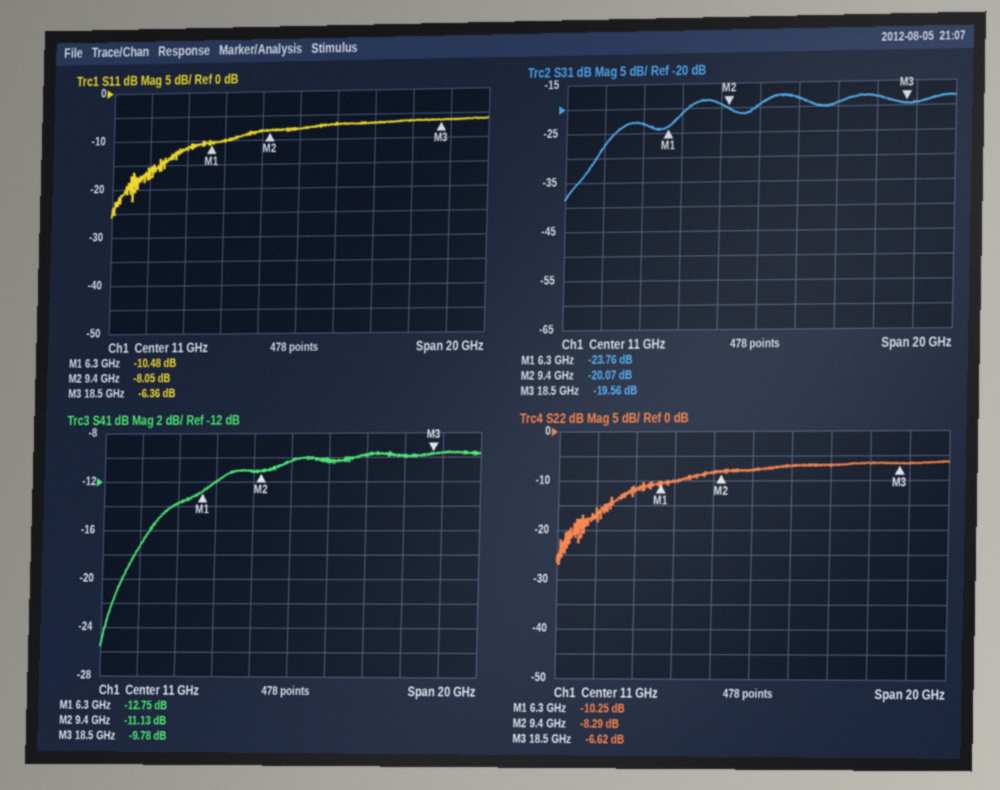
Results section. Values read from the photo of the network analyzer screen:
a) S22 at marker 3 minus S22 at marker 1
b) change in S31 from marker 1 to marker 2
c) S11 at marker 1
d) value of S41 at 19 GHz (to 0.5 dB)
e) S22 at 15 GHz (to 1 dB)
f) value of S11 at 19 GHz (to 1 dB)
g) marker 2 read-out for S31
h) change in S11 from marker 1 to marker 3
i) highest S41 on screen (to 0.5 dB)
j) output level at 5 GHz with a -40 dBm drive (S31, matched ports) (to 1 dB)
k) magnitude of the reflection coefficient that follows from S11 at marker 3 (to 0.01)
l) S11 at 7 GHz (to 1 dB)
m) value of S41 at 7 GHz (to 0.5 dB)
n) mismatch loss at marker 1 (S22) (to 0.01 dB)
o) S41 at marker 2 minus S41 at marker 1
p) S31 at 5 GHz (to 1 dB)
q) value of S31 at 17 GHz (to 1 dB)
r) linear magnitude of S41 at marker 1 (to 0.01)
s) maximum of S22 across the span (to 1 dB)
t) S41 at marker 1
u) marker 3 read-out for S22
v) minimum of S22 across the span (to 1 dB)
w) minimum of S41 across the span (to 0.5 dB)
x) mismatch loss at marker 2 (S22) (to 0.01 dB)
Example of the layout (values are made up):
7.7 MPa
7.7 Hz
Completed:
3.63 dB
3.69 dB
-10.48 dB
-9.5 dB
-7 dB
-6 dB
-20.07 dB
4.12 dB
-9.5 dB
-63 dBm
0.48
-10 dB
-12.0 dB
0.43 dB
1.62 dB
-23 dB
-18 dB
0.23
-6 dB
-12.75 dB
-6.62 dB
-27 dB
-25.5 dB
0.70 dB
